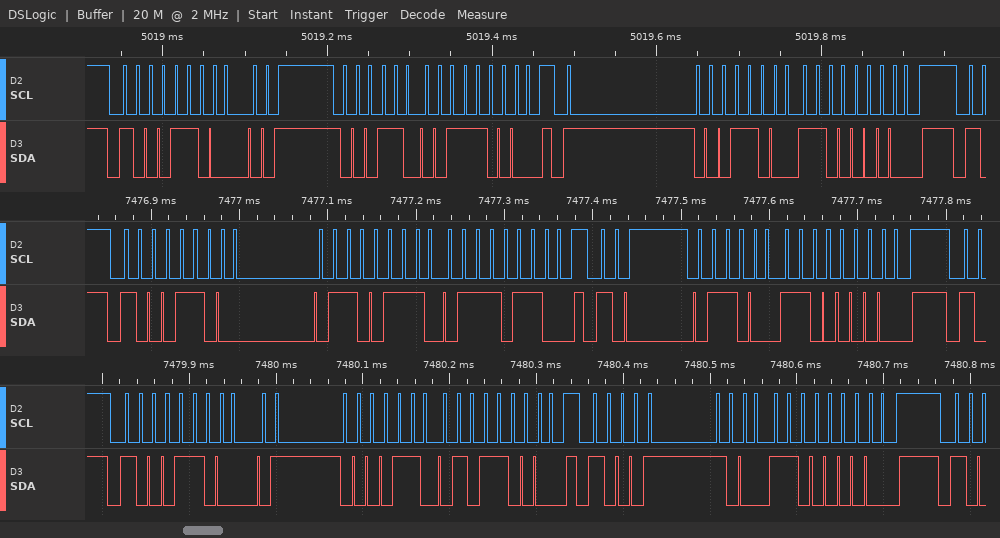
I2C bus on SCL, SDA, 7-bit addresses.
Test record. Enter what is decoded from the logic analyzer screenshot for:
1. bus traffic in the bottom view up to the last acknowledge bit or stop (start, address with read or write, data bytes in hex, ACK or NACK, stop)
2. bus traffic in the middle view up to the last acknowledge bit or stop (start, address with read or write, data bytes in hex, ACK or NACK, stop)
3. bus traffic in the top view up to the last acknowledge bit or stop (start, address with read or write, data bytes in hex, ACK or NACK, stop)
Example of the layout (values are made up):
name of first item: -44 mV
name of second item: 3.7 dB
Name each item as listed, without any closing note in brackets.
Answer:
bus traffic in the bottom view up to the last acknowledge bit or stop: start, address 46 write ACK, 43 ACK, 58 ACK, stop, start, address 46 write ACK, C0 ACK, stop
bus traffic in the middle view up to the last acknowledge bit or stop: start, address 46 write ACK, 67 ACK, 76 ACK, stop, start, address 46 write ACK, C0 ACK, stop
bus traffic in the top view up to the last acknowledge bit or stop: start, address 46 write ACK, 23 ACK, 38 ACK, stop, start, address 46 write ACK, C0 ACK, stop
